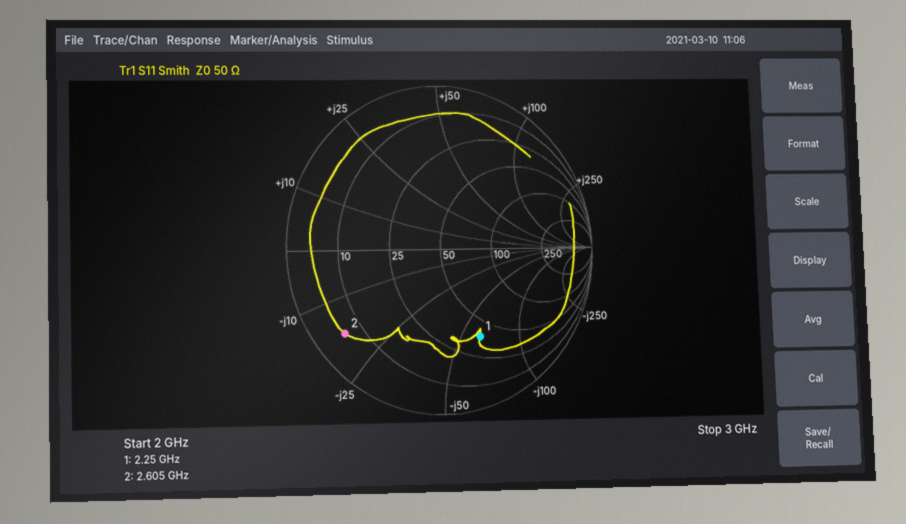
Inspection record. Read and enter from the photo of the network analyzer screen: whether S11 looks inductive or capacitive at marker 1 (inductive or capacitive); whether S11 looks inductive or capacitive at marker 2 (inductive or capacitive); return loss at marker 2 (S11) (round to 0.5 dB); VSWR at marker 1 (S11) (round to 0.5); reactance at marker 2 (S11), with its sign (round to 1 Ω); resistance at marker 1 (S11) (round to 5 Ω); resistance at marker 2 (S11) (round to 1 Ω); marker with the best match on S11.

capacitive
capacitive
2.0 dB
4.0
-17 Ω
40 Ω
6 Ω
marker 1
